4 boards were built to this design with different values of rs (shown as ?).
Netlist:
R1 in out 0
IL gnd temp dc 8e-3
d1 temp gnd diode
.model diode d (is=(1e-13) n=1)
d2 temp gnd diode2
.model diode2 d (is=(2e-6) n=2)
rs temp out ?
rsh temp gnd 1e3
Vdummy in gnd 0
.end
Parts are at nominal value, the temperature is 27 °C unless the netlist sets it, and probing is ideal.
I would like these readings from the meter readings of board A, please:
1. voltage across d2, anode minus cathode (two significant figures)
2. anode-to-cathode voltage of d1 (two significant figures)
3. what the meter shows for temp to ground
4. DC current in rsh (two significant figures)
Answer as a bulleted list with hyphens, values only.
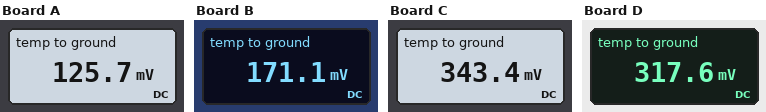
- 130 mV
- 130 mV
- 125.7 mV
- 130 µA
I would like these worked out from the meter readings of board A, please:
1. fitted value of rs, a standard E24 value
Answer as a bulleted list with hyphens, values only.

- 16 Ω
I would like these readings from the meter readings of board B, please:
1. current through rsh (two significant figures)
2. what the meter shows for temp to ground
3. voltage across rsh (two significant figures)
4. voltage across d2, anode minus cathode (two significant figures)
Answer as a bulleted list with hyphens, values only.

- 170 µA
- 171.1 mV
- 170 mV
- 170 mV
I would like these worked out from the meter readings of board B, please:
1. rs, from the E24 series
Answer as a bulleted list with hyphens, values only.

- 22 Ω
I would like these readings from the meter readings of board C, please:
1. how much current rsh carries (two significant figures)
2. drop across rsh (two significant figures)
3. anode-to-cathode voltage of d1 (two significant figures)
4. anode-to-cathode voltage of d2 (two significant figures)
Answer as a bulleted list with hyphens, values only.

- 340 µA
- 340 mV
- 340 mV
- 340 mV
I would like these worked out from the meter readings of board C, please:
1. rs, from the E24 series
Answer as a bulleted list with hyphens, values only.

- 56 Ω
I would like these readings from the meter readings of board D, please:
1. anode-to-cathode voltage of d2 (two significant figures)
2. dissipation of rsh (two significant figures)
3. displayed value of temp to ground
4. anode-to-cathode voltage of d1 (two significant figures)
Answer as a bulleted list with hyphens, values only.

- 320 mV
- 100 µW
- 317.6 mV
- 320 mV
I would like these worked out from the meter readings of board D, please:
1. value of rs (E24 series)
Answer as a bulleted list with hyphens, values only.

- 47 Ω
